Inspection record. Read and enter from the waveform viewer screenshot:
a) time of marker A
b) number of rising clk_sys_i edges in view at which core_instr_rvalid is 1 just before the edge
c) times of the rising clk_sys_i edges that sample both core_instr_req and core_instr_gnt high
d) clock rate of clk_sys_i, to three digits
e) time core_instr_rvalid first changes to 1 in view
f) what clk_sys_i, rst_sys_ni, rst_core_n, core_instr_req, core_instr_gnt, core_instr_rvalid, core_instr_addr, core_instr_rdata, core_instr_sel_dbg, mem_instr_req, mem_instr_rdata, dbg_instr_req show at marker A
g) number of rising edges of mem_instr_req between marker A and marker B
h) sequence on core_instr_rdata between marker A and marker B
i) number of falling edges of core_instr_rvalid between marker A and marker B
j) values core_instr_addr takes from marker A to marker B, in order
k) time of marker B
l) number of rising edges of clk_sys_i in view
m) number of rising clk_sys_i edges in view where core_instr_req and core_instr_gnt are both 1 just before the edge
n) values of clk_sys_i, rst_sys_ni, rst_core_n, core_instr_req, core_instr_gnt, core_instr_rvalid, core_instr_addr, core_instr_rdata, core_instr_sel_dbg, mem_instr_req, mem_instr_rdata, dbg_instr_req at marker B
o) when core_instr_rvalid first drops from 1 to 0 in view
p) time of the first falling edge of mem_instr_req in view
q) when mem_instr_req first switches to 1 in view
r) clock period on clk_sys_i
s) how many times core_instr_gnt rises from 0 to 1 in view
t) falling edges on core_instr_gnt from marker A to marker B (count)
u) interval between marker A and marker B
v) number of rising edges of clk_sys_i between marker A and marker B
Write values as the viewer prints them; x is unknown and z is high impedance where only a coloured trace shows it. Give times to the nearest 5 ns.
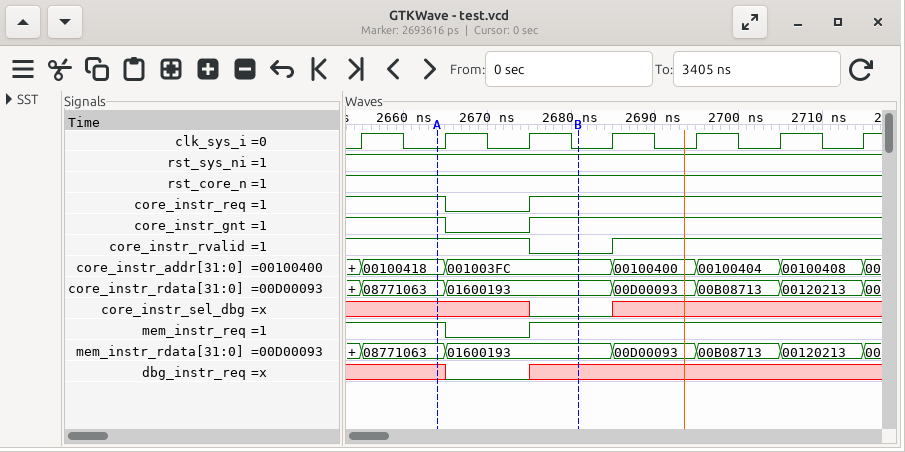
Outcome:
2665 ns
6
2655 ns, 2665 ns, 2685 ns, 2695 ns, 2705 ns, 2715 ns
100 MHz
2685 ns
clk_sys_i=0, rst_sys_ni=1, rst_core_n=1, core_instr_req=1, core_instr_gnt=1, core_instr_rvalid=1, core_instr_addr=00100418, core_instr_rdata=08771063, core_instr_sel_dbg=x, mem_instr_req=1, mem_instr_rdata=08771063, dbg_instr_req=x
1
08771063, 01600193
1
00100418, 001003FC
2680 ns
7
6
clk_sys_i=0, rst_sys_ni=1, rst_core_n=1, core_instr_req=1, core_instr_gnt=1, core_instr_rvalid=0, core_instr_addr=001003FC, core_instr_rdata=01600193, core_instr_sel_dbg=0, mem_instr_req=1, mem_instr_rdata=01600193, dbg_instr_req=x
2675 ns
2665 ns
2675 ns
10 ns
1
1
15 ns
2
